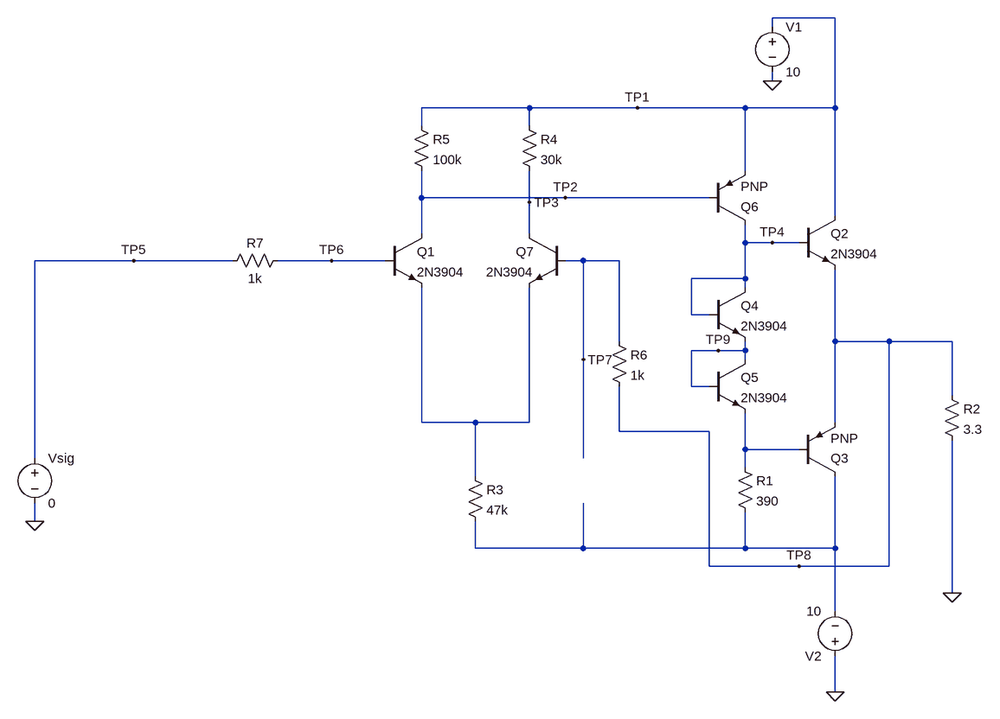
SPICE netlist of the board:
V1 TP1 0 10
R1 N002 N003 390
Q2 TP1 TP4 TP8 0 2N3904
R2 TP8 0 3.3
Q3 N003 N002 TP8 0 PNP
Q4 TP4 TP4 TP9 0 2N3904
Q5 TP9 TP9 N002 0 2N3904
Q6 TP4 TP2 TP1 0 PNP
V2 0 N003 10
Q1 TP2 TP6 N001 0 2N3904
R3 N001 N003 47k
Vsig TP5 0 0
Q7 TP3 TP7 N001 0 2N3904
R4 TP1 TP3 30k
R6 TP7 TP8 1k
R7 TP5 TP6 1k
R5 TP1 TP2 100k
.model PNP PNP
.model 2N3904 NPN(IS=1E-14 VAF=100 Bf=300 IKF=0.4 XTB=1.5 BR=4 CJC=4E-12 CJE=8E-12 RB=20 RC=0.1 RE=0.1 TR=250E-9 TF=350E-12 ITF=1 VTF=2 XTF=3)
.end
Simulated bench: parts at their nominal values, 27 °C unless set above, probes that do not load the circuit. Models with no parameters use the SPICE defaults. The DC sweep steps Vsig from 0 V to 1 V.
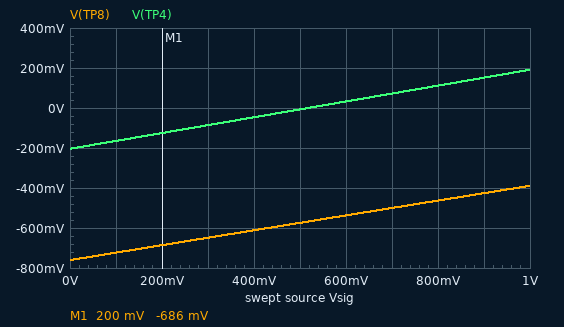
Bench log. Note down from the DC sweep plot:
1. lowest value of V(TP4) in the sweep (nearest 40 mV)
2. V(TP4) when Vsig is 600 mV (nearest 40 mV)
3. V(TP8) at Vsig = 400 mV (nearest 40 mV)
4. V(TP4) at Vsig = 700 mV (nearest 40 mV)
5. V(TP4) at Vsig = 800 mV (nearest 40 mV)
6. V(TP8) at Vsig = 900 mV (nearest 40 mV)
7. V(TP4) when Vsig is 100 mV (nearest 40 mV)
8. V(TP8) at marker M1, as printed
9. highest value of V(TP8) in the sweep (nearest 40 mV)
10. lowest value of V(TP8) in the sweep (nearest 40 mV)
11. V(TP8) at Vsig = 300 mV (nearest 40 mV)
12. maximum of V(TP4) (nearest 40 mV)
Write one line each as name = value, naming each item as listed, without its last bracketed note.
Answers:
lowest value of V(TP4) in the sweep = -200 mV
V(TP4) when Vsig is 600 mV = 40 mV
V(TP8) at Vsig = 400 mV = -600 mV
V(TP4) at Vsig = 700 mV = 80 mV
V(TP4) at Vsig = 800 mV = 120 mV
V(TP8) at Vsig = 900 mV = -440 mV
V(TP4) when Vsig is 100 mV = -160 mV
V(TP8) at marker M1, as printed = -686 mV
highest value of V(TP8) in the sweep = -400 mV
lowest value of V(TP8) in the sweep = -760 mV
V(TP8) at Vsig = 300 mV = -640 mV
maximum of V(TP4) = 200 mV
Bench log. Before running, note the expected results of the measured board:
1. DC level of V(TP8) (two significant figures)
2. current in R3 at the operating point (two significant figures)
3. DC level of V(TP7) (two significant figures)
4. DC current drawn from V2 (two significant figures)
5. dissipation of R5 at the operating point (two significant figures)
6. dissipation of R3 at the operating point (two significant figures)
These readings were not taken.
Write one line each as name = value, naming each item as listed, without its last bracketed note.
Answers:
DC level of V(TP8) = -760 mV
current in R3 at the operating point = 200 µA
DC level of V(TP7) = -760 mV
DC current drawn from V2 = 250 mA
dissipation of R5 at the operating point = 7.2 µW
dissipation of R3 at the operating point = 1.9 mW
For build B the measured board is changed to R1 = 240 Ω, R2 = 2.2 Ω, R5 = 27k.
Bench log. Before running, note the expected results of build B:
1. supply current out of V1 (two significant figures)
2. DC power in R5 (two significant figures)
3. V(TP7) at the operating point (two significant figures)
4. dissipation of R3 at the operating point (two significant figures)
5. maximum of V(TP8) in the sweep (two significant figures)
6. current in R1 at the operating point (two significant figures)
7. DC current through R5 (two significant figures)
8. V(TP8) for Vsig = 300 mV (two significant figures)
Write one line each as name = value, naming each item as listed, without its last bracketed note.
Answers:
supply current out of V1 = 17 mA
DC power in R5 = 27 µW
V(TP7) at the operating point = -2.4 V
dissipation of R3 at the operating point = 1.9 mW
maximum of V(TP8) in the sweep = -2.2 V
current in R1 at the operating point = 28 mA
DC current through R5 = 31 µA
V(TP8) for Vsig = 300 mV = -2.3 V
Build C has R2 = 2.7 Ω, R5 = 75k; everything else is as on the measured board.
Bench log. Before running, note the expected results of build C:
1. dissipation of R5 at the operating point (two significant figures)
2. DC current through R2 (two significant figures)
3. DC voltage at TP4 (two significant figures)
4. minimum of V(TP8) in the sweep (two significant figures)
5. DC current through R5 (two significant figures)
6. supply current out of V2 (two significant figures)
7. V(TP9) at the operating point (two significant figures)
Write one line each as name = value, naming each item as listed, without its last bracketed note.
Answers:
dissipation of R5 at the operating point = 9.6 µW
DC current through R2 = 270 mA
DC voltage at TP4 = -170 mV
minimum of V(TP8) in the sweep = -720 mV
DC current through R5 = 11 µA
supply current out of V2 = 290 mA
V(TP9) at the operating point = -910 mV
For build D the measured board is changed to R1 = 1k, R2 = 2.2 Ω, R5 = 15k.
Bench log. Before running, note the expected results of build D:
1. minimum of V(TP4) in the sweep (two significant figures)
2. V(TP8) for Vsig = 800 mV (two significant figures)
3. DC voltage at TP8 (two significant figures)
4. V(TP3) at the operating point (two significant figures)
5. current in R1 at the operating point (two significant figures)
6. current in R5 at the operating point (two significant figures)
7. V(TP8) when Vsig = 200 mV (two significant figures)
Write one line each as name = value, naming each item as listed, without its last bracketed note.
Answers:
minimum of V(TP4) in the sweep = 560 mV
V(TP8) for Vsig = 800 mV = 760 mV
DC voltage at TP8 = -26 mV
V(TP3) at the operating point = 8.4 V
current in R1 at the operating point = 9.1 mA
current in R5 at the operating point = 55 µA
V(TP8) when Vsig = 200 mV = 170 mV
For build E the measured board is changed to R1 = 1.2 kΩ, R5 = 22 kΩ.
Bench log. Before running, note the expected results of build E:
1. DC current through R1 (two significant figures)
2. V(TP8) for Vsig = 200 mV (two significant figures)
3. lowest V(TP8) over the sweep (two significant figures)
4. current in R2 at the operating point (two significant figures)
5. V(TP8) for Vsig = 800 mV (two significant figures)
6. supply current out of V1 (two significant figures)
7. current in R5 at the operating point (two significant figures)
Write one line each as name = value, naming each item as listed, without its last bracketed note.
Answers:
DC current through R1 = 7.7 mA
V(TP8) for Vsig = 200 mV = 190 mV
lowest V(TP8) over the sweep = -7.1 mV
current in R2 at the operating point = 2.2 mA
V(TP8) for Vsig = 800 mV = 790 mV
supply current out of V1 = 8.1 mA
current in R5 at the operating point = 38 µA
